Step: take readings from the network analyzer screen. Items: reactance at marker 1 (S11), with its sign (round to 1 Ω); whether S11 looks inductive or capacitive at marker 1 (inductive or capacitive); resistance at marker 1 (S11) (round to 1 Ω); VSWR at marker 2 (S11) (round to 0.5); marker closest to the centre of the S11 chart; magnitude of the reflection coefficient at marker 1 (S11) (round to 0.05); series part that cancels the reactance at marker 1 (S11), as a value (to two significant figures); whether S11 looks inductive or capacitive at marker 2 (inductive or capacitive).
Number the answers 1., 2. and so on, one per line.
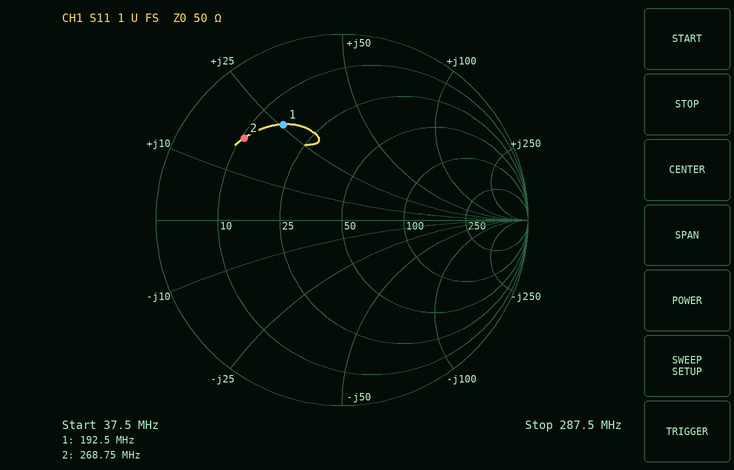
1. +26 Ω
2. inductive
3. 16 Ω
4. 5.5
5. marker 1
6. 0.60
7. 32 pF
8. inductive
